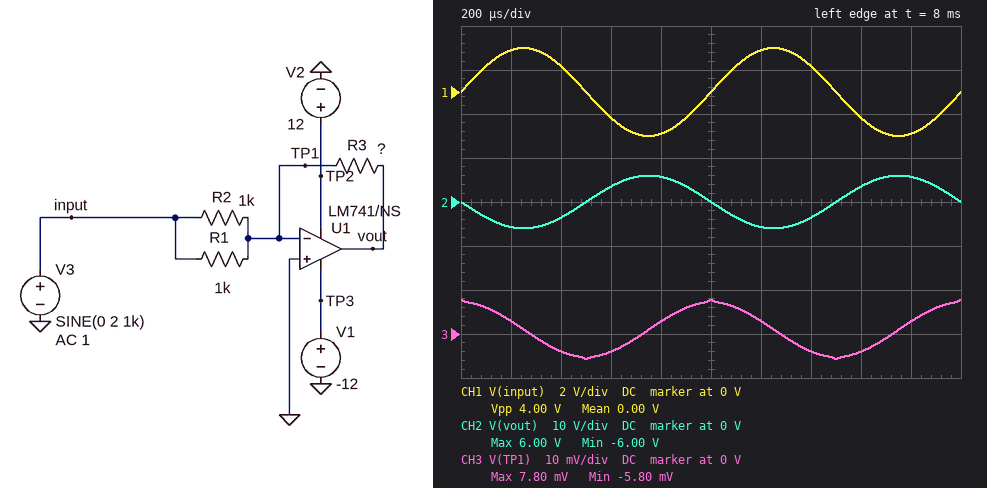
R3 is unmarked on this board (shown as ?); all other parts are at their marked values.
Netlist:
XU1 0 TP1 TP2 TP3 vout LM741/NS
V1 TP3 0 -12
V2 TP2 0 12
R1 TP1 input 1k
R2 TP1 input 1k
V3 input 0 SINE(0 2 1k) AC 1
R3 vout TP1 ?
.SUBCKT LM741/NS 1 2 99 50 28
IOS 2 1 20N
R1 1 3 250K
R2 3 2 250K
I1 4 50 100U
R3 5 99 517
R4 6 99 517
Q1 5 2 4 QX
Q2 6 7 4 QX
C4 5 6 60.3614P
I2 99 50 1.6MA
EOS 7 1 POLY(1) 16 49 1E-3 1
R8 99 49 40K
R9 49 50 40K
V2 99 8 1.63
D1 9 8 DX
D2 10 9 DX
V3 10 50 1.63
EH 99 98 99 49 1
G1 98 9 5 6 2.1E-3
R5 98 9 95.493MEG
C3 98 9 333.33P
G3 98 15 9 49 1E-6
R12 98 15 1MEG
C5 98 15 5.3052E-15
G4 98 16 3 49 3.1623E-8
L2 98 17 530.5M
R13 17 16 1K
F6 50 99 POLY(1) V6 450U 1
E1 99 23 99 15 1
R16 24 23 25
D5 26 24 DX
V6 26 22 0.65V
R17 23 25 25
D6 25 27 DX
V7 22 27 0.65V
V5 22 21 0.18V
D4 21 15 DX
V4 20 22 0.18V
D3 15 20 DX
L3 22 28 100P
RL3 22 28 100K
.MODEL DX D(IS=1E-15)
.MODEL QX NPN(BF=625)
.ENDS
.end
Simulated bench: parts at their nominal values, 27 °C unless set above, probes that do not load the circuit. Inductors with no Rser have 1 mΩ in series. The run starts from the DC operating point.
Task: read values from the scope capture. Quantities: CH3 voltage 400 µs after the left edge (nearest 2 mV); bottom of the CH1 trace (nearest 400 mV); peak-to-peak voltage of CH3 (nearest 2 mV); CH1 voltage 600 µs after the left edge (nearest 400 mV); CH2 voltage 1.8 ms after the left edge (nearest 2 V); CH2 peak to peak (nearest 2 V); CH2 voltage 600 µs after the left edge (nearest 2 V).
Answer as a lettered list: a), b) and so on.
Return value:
a) -4 mV
b) -2.0 V
c) 14 mV
d) -1.2 V
e) 6 V
f) 12 V
g) 4 V
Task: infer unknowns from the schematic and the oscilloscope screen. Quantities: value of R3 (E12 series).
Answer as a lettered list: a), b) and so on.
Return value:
a) 1.5 kΩ
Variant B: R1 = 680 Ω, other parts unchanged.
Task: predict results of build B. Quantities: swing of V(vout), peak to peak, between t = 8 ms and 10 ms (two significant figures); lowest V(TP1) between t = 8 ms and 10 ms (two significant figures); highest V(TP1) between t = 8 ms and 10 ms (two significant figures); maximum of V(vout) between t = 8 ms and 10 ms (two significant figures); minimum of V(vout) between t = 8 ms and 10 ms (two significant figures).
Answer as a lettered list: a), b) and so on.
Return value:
a) 15 V
b) -7.4 mV
c) 9.4 mV
d) 7.4 V
e) -7.4 V
